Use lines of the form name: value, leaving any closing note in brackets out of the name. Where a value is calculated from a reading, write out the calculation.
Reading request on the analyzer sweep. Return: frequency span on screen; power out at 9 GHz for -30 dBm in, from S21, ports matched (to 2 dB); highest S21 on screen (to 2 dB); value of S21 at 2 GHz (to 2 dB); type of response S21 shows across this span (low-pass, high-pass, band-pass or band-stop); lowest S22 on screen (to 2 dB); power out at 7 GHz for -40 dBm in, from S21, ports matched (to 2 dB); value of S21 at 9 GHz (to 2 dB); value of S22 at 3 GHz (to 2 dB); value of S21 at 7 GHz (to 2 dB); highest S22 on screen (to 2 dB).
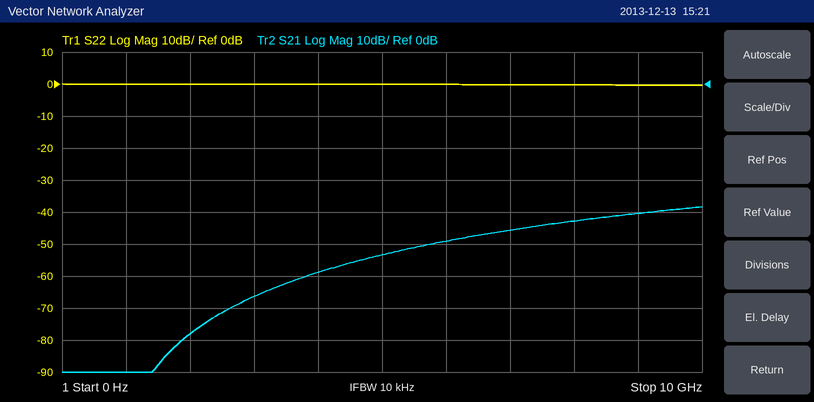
frequency span on screen: 10 GHz
power out at 9 GHz for -30 dBm in, from S21, ports matched: -30 dBm + (-40 dB) = -70 dBm
highest S21 on screen: -38 dB
value of S21 at 2 GHz: -78 dB
type of response S21 shows across this span: high-pass
lowest S22 on screen: 0 dB
power out at 7 GHz for -40 dBm in, from S21, ports matched: -40 dBm + (-46 dB) = -86 dBm
value of S21 at 9 GHz: -40 dB
value of S22 at 3 GHz: 0 dB
value of S21 at 7 GHz: -46 dB
highest S22 on screen: 0 dB
